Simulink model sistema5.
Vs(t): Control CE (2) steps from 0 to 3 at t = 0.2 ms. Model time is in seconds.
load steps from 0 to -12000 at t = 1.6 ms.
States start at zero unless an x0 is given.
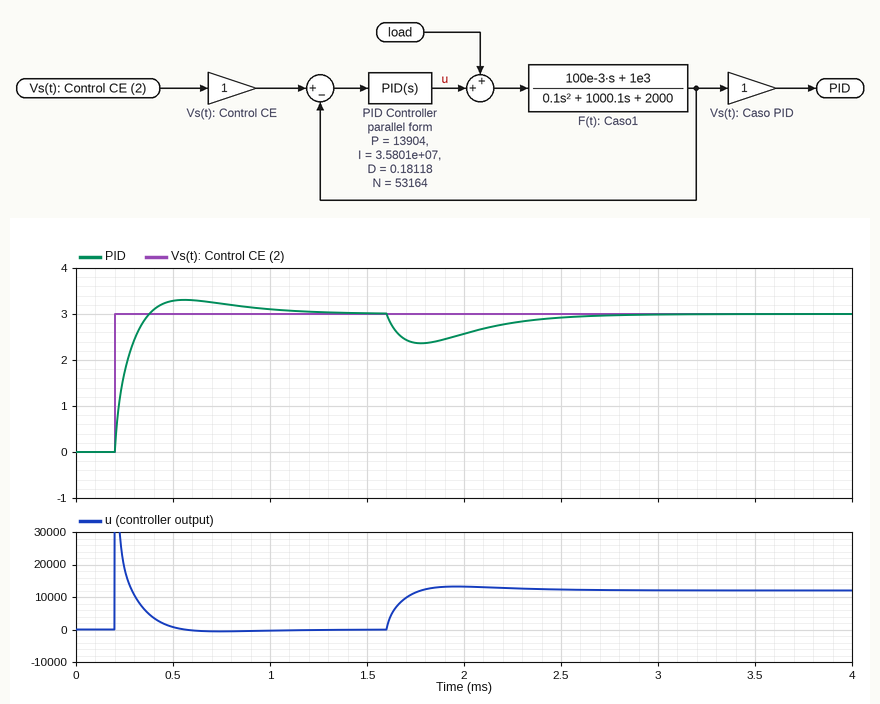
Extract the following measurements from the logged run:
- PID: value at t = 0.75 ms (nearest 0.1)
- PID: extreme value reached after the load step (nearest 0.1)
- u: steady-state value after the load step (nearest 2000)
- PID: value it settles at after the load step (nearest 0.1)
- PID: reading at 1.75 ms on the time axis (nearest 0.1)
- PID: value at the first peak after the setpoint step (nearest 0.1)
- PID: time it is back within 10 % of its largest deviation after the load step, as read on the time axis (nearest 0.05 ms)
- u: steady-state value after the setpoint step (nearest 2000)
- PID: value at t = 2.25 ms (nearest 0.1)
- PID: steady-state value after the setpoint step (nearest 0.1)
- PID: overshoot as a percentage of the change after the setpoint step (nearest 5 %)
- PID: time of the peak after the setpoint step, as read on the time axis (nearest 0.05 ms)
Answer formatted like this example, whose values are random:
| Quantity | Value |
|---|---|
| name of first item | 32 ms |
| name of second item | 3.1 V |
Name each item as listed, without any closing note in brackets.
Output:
| Quantity | Value |
|---|---|
| PID: value at t = 0.75 ms | 3.2 |
| PID: extreme value reached after the load step | 2.4 |
| u: steady-state value after the load step | 12000 |
| PID: value it settles at after the load step | 3.0 |
| PID: reading at 1.75 ms on the time axis | 2.4 |
| PID: value at the first peak after the setpoint step | 3.3 |
| PID: time it is back within 10 % of its largest deviation after the load step, as read on the time axis | 2.55 ms |
| u: steady-state value after the setpoint step | 0 |
| PID: value at t = 2.25 ms | 2.8 |
| PID: steady-state value after the setpoint step | 3.0 |
| PID: overshoot as a percentage of the change after the setpoint step | 10 % |
| PID: time of the peak after the setpoint step, as read on the time axis | 0.55 ms |
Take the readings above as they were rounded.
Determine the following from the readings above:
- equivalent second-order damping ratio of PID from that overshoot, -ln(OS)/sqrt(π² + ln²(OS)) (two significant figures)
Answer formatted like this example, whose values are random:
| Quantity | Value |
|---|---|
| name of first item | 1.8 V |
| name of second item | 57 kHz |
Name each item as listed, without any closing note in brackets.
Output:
| Quantity | Value |
|---|---|
| equivalent second-order damping ratio of PID from that overshoot, -ln(OS)/sqrt(π² + ln²(OS)) | 0.59 |
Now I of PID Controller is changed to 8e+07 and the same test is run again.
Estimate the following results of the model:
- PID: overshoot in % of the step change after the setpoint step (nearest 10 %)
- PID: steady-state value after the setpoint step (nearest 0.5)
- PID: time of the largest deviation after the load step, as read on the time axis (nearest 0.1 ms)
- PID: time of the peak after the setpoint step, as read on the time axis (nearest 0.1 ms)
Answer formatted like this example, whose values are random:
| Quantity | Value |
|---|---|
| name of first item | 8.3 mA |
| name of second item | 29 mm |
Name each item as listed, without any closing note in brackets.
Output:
| Quantity | Value |
|---|---|
| PID: overshoot in % of the step change after the setpoint step | 20 % |
| PID: steady-state value after the setpoint step | 3.0 |
| PID: time of the largest deviation after the load step, as read on the time axis | 1.7 ms |
| PID: time of the peak after the setpoint step, as read on the time axis | 0.5 ms |
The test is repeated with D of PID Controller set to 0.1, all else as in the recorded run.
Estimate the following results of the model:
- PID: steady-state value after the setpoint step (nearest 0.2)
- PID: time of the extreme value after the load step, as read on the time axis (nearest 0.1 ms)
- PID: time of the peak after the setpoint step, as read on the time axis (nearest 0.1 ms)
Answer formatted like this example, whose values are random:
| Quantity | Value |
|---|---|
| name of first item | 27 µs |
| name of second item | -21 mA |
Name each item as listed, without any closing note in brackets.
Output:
| Quantity | Value |
|---|---|
| PID: steady-state value after the setpoint step | 3.0 |
| PID: time of the extreme value after the load step, as read on the time axis | 1.8 ms |
| PID: time of the peak after the setpoint step, as read on the time axis | 0.5 ms |
